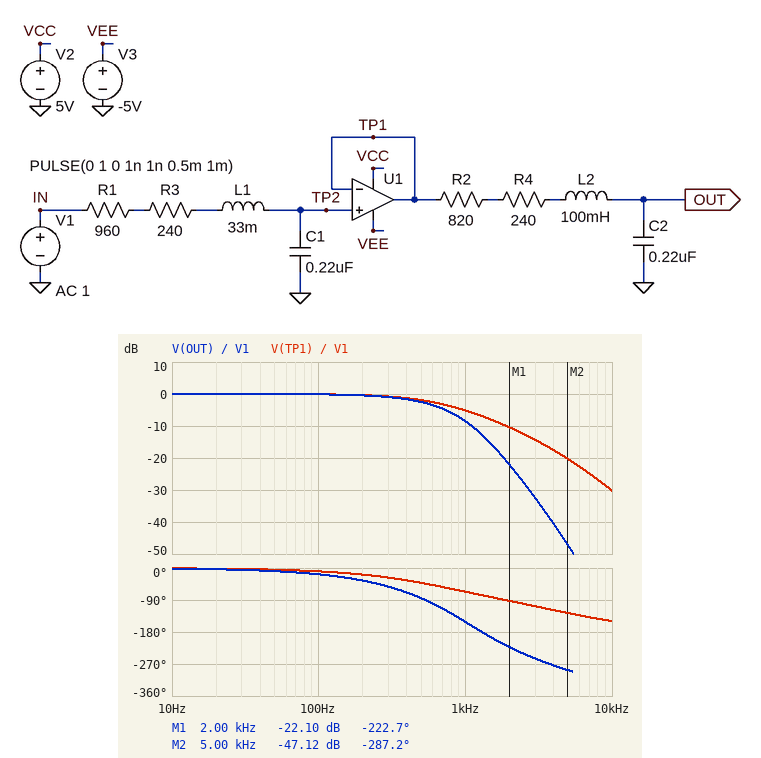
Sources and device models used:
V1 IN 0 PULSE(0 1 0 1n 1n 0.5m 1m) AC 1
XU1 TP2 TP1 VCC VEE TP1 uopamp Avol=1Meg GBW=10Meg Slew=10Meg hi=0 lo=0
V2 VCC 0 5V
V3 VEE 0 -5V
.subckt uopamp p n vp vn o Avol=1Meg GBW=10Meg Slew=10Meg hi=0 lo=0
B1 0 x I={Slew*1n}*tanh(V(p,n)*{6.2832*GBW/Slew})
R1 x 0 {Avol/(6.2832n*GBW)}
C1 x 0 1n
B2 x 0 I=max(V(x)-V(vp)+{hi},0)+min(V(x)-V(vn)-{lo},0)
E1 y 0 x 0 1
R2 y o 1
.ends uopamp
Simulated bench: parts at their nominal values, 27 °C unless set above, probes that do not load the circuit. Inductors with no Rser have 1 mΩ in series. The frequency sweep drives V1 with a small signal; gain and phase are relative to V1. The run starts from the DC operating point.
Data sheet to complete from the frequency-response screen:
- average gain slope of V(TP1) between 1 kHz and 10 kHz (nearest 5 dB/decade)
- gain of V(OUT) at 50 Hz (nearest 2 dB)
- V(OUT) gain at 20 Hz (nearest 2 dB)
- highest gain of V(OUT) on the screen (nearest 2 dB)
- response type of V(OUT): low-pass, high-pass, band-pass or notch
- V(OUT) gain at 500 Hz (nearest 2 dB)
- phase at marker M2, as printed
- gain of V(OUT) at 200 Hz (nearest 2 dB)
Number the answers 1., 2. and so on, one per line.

1. -25 dB/decade
2. 0 dB
3. 0 dB
4. 0 dB
5. low-pass
6. -2 dB
7. -287.2 deg
8. 0 dB
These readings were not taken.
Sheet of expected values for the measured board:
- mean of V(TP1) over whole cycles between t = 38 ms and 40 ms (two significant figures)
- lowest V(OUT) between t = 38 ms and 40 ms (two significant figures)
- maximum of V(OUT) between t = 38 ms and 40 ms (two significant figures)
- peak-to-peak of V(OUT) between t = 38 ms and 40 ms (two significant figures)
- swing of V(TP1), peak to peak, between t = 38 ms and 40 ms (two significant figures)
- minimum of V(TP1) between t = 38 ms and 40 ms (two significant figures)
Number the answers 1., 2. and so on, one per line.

1. 500 mV
2. 260 mV
3. 740 mV
4. 490 mV
5. 760 mV
6. 120 mV
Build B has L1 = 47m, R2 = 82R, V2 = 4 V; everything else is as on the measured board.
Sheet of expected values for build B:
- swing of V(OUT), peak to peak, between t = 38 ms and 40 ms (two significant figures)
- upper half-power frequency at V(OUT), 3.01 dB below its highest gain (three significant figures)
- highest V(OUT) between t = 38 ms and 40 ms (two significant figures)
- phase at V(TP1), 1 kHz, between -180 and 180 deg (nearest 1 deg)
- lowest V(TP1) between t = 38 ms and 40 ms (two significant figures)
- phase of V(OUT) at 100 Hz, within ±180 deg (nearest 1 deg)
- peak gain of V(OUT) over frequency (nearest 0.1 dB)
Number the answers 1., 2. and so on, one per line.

1. 1.6 V
2. 1.18 kHz
3. 1.3 V
4. -70 deg
5. 110 mV
6. -12 deg
7. 1.9 dB
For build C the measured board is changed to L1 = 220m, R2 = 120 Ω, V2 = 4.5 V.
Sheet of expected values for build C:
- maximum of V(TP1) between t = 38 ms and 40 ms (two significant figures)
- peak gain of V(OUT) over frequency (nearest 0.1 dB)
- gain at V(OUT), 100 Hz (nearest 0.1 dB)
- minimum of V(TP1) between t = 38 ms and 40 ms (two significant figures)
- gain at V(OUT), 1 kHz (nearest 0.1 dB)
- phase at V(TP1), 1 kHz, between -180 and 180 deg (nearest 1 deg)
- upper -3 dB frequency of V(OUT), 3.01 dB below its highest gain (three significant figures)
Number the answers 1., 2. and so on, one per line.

1. 850 mV
2. 2.2 dB
3. 0.1 dB
4. 150 mV
5. 0.2 dB
6. -119 deg
7. 1.06 kHz
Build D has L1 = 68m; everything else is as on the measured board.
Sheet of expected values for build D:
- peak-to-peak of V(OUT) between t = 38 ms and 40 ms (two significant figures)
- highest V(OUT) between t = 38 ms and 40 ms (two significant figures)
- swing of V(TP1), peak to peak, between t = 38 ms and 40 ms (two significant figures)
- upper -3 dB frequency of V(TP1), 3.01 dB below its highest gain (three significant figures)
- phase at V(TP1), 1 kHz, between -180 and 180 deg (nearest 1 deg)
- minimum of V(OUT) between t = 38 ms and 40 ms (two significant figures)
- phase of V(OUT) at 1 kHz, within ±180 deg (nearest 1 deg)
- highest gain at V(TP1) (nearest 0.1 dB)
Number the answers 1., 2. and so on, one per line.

1. 510 mV
2. 760 mV
3. 790 mV
4. 752 Hz
5. -76 deg
6. 240 mV
7. -161 deg
8. 0 dB
